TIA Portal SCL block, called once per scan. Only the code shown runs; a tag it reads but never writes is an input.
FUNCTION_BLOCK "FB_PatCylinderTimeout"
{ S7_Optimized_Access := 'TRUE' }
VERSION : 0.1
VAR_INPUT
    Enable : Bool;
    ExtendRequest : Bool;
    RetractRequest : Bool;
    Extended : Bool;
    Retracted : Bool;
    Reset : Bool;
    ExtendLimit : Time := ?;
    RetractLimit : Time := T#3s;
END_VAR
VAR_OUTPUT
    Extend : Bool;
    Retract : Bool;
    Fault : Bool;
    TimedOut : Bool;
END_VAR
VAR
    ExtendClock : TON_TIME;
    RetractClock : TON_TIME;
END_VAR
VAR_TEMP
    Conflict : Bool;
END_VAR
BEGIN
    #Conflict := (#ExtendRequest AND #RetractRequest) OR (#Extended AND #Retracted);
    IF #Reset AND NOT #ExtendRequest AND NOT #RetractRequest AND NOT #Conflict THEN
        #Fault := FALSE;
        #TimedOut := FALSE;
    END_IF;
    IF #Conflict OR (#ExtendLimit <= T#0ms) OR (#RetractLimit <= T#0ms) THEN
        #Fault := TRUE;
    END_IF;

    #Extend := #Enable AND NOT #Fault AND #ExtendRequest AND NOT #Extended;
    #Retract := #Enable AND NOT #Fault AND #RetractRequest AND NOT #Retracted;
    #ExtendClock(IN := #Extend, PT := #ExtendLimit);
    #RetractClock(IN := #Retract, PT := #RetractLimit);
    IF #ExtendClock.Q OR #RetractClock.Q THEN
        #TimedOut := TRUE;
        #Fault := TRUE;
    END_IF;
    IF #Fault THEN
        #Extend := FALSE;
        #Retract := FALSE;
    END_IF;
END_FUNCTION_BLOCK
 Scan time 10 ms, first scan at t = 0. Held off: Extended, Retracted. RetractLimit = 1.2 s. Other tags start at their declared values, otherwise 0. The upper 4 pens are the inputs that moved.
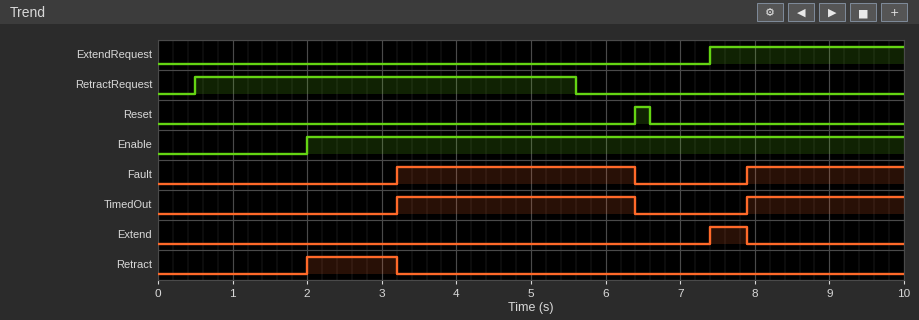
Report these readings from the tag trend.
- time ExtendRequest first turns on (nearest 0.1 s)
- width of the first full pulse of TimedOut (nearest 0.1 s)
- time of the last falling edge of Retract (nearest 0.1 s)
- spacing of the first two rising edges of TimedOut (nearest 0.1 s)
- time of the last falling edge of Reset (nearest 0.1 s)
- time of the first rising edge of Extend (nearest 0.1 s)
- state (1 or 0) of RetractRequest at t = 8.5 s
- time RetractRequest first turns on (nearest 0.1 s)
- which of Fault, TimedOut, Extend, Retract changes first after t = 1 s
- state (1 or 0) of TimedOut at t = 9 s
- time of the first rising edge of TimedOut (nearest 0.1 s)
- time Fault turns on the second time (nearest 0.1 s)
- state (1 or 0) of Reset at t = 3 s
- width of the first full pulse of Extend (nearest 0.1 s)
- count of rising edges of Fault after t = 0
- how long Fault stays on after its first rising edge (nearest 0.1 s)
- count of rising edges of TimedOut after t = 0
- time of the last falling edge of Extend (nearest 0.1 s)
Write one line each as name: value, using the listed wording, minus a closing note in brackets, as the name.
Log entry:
time ExtendRequest first turns on: 7.4 s
width of the first full pulse of TimedOut: 3.2 s
time of the last falling edge of Retract: 3.2 s
spacing of the first two rising edges of TimedOut: 4.7 s
time of the last falling edge of Reset: 6.6 s
time of the first rising edge of Extend: 7.4 s
state (1 or 0) of RetractRequest at t = 8.5 s: 0
time RetractRequest first turns on: 0.5 s
which of Fault, TimedOut, Extend, Retract changes first after t = 1 s: Retract
state (1 or 0) of TimedOut at t = 9 s: 1
time of the first rising edge of TimedOut: 3.2 s
time Fault turns on the second time: 7.9 s
state (1 or 0) of Reset at t = 3 s: 0
width of the first full pulse of Extend: 0.5 s
count of rising edges of Fault after t = 0: 2
how long Fault stays on after its first rising edge: 3.2 s
count of rising edges of TimedOut after t = 0: 2
time of the last falling edge of Extend: 7.9 s
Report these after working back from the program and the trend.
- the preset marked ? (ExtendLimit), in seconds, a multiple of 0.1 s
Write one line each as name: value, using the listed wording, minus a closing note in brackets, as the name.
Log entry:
the preset marked ? (ExtendLimit), in seconds, a multiple of 0.1 s: 0.5 s
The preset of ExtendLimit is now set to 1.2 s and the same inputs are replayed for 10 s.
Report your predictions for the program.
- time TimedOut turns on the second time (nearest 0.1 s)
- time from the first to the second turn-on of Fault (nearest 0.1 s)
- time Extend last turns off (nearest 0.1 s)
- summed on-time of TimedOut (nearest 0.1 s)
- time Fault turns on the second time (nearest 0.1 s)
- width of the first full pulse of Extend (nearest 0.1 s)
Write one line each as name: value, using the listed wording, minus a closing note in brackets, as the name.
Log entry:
time TimedOut turns on the second time: 8.6 s
time from the first to the second turn-on of Fault: 5.4 s
time Extend last turns off: 8.6 s
summed on-time of TimedOut: 4.6 s
time Fault turns on the second time: 8.6 s
width of the first full pulse of Extend: 1.2 s
